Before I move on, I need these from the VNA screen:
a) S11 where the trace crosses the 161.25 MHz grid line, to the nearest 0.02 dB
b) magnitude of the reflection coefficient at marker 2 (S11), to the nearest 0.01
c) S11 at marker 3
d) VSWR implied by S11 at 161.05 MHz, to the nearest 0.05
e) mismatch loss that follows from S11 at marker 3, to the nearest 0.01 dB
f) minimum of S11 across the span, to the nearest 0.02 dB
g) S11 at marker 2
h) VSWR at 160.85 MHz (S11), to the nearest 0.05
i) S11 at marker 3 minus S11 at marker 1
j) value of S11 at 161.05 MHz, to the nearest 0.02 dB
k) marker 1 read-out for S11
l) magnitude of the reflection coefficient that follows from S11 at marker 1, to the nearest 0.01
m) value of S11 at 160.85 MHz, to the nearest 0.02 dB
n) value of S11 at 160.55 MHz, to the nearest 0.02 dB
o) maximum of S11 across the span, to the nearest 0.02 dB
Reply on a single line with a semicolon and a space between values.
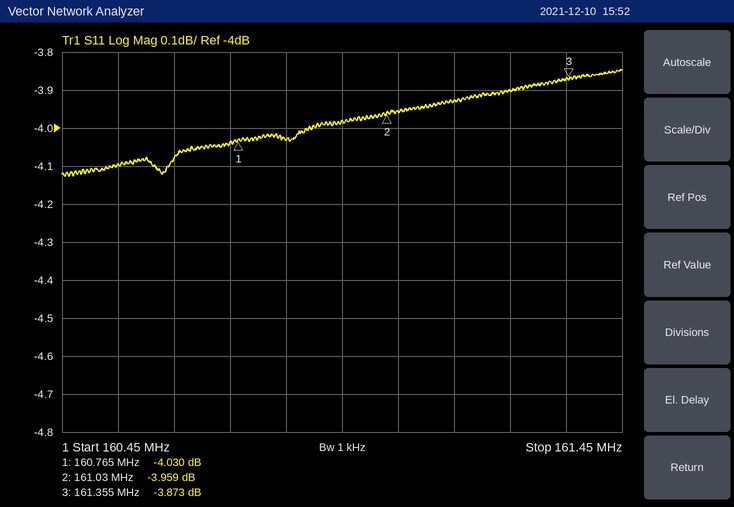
-3.90 dB; 0.63; -3.873 dB; 4.45; 2.29 dB; -4.12 dB; -3.959 dB; 4.40; 0.157 dB; -3.96 dB; -4.030 dB; 0.63; -4.04 dB; -4.10 dB; -3.84 dB
